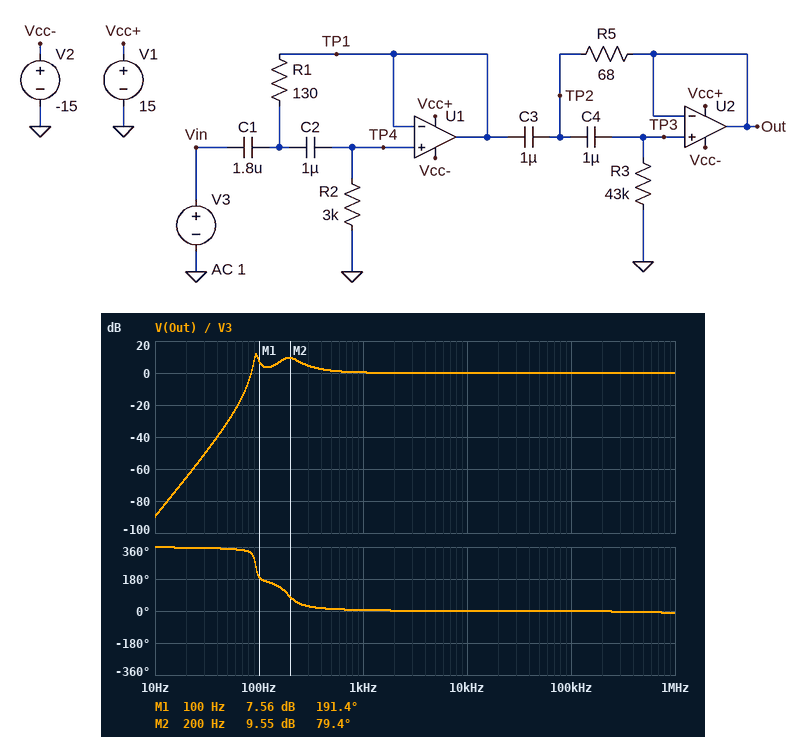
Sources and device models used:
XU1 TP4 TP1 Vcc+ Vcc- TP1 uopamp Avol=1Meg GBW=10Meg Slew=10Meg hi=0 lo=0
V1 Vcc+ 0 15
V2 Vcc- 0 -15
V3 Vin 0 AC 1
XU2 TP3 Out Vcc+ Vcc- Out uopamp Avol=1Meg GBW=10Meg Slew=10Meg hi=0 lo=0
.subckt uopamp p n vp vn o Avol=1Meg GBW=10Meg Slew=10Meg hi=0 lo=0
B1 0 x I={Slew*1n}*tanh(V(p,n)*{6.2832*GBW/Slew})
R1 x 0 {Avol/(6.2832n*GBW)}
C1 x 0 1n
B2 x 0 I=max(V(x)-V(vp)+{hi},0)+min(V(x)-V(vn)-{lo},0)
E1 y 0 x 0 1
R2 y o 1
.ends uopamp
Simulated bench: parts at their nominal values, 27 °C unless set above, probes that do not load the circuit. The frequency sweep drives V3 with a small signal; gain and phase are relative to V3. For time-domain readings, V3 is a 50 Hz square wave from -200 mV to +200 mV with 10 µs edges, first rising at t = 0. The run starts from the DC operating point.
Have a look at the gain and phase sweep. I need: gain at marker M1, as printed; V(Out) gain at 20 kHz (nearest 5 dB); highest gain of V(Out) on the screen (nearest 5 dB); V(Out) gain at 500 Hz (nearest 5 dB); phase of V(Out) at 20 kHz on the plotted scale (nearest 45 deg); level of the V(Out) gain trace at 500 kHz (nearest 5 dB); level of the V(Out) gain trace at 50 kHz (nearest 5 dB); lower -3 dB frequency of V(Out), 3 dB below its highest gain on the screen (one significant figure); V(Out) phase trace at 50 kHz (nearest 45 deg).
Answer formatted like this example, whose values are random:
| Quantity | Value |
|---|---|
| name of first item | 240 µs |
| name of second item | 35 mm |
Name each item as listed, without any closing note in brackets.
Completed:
| Quantity | Value |
|---|---|
| gain at marker M1, as printed | 7.56 dB |
| V(Out) gain at 20 kHz | 0 dB |
| highest gain of V(Out) on the screen | 10 dB |
| V(Out) gain at 500 Hz | 0 dB |
| phase of V(Out) at 20 kHz on the plotted scale | 0 deg |
| level of the V(Out) gain trace at 500 kHz | 0 dB |
| level of the V(Out) gain trace at 50 kHz | 0 dB |
| lower -3 dB frequency of V(Out), 3 dB below its highest gain on the screen | 90 Hz |
| V(Out) phase trace at 50 kHz | 0 deg |
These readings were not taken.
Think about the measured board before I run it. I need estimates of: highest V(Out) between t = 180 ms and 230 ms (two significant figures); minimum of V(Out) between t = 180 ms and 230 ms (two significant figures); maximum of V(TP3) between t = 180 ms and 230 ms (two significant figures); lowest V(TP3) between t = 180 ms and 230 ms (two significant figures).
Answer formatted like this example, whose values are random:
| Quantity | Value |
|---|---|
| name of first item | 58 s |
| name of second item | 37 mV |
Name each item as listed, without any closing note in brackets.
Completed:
| Quantity | Value |
|---|---|
| highest V(Out) between t = 180 ms and 230 ms | 420 mV |
| minimum of V(Out) between t = 180 ms and 230 ms | -420 mV |
| maximum of V(TP3) between t = 180 ms and 230 ms | 420 mV |
| lowest V(TP3) between t = 180 ms and 230 ms | -420 mV |
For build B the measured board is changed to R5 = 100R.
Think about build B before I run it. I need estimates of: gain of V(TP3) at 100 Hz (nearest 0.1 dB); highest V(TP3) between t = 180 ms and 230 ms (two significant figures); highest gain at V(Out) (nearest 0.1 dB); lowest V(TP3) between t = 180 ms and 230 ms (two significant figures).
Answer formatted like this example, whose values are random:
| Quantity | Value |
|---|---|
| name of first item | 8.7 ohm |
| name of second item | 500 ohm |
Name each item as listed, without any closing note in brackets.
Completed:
| Quantity | Value |
|---|---|
| gain of V(TP3) at 100 Hz | -1.2 dB |
| highest V(TP3) between t = 180 ms and 230 ms | 400 mV |
| highest gain at V(Out) | 8.9 dB |
| lowest V(TP3) between t = 180 ms and 230 ms | -400 mV |
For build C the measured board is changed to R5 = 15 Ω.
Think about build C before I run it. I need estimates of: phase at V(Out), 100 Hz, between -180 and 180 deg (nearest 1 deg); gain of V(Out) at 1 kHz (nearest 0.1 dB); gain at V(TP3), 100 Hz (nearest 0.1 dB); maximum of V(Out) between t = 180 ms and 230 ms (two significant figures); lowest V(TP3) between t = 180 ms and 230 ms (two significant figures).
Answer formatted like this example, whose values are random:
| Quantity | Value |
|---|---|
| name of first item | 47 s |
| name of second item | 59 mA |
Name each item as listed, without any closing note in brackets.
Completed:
| Quantity | Value |
|---|---|
| phase at V(Out), 100 Hz, between -180 and 180 deg | -19 deg |
| gain of V(Out) at 1 kHz | 0.6 dB |
| gain at V(TP3), 100 Hz | -18.1 dB |
| maximum of V(Out) between t = 180 ms and 230 ms | 380 mV |
| lowest V(TP3) between t = 180 ms and 230 ms | -380 mV |
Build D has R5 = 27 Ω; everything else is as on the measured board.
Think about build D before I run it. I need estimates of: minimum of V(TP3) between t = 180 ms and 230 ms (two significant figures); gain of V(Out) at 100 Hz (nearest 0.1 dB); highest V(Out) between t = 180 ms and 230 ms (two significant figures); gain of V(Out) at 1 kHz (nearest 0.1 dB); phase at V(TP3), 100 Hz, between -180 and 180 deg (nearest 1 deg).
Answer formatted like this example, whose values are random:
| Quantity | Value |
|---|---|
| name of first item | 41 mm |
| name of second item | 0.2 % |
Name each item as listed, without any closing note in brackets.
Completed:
| Quantity | Value |
|---|---|
| minimum of V(TP3) between t = 180 ms and 230 ms | -1.9 V |
| gain of V(Out) at 100 Hz | -10.2 dB |
| highest V(Out) between t = 180 ms and 230 ms | 1.9 V |
| gain of V(Out) at 1 kHz | 0.5 dB |
| phase at V(TP3), 100 Hz, between -180 and 180 deg | -21 deg |
